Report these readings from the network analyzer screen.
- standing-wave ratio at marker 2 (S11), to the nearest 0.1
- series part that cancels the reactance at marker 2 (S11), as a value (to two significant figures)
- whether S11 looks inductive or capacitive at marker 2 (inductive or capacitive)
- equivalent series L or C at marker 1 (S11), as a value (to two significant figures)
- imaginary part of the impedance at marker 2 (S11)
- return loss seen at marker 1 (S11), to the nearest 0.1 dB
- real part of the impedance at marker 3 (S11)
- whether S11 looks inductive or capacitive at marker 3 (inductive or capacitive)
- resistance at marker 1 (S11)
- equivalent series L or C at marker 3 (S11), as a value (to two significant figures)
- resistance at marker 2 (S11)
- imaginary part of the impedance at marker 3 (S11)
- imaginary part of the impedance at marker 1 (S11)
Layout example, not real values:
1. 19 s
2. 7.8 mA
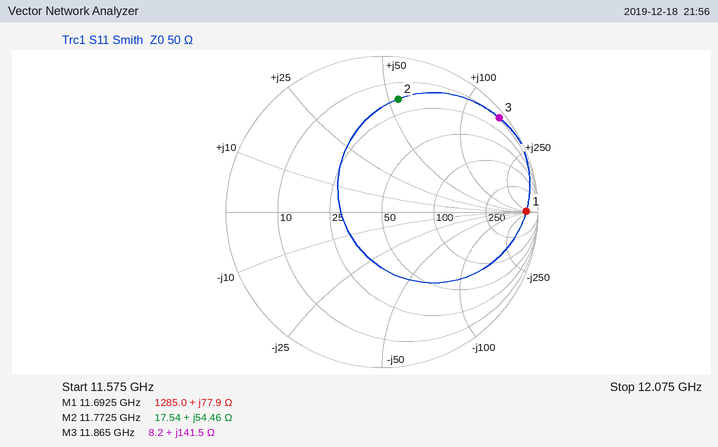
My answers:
1. 6.4
2. 250 fF
3. inductive
4. 1.1 nH
5. +54.46 Ω
6. 0.7 dB
7. 8.2 Ω
8. inductive
9. 1285.0 Ω
10. 1.9 nH
11. 17.54 Ω
12. +141.5 Ω
13. +77.9 Ω
